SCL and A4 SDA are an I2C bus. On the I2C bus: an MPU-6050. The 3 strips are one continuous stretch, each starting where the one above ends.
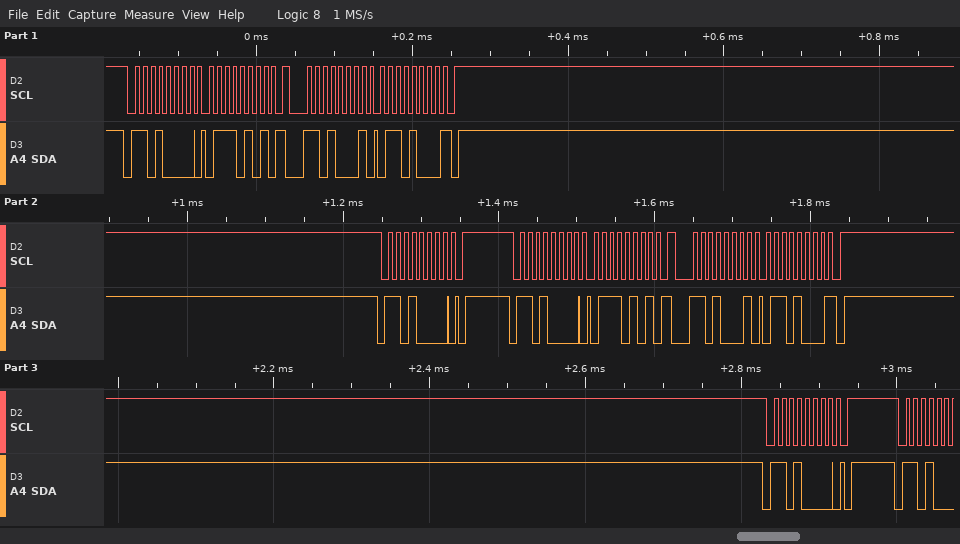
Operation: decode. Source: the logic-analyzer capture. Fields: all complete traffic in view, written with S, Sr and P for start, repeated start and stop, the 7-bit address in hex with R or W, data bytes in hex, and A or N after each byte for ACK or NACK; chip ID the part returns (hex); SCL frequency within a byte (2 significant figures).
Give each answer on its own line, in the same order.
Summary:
S 68W A 75 A Sr 68R A 68 N P S 68W A P S 68W A 75 A Sr 68R A 68 N P S 68W A P
0x68
100 kHz
